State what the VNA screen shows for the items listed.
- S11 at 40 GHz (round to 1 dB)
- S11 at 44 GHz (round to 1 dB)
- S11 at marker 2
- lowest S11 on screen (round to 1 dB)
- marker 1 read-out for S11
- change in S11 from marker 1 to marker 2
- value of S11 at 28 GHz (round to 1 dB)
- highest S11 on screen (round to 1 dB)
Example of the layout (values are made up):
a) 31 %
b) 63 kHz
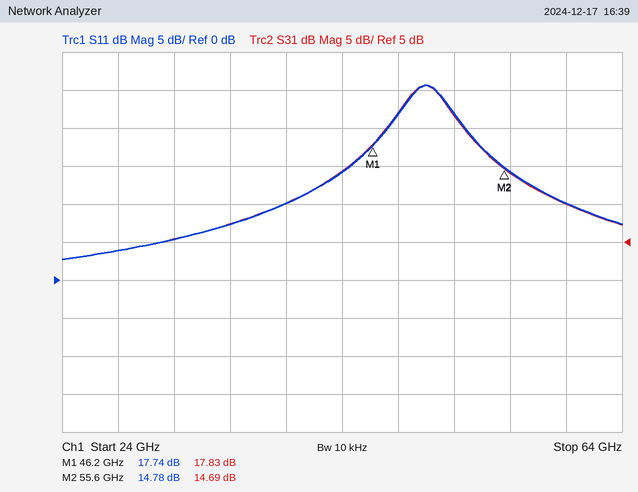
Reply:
a) 10 dB
b) 14 dB
c) 14.78 dB
d) 3 dB
e) 17.74 dB
f) -2.96 dB
g) 4 dB
h) 26 dB
